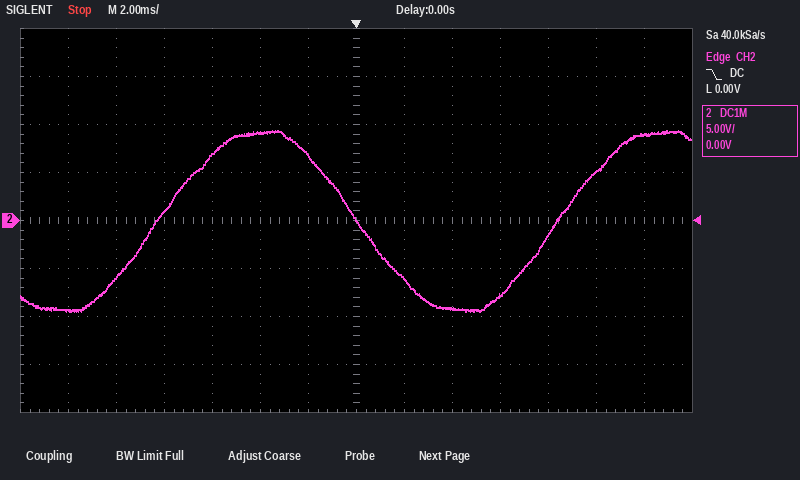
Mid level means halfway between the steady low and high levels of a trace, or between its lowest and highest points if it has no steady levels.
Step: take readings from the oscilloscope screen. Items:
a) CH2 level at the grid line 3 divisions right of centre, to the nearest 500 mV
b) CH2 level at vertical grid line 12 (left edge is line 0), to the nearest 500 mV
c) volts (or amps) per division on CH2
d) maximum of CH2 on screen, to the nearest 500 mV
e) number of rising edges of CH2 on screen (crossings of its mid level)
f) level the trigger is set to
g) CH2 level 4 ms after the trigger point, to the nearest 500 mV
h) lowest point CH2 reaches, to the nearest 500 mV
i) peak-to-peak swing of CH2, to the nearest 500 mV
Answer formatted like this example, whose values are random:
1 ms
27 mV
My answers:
-8.0 V
5.0 V
5 V
9.5 V
2
0.00 V
-9.0 V
-9.5 V
19.0 V
